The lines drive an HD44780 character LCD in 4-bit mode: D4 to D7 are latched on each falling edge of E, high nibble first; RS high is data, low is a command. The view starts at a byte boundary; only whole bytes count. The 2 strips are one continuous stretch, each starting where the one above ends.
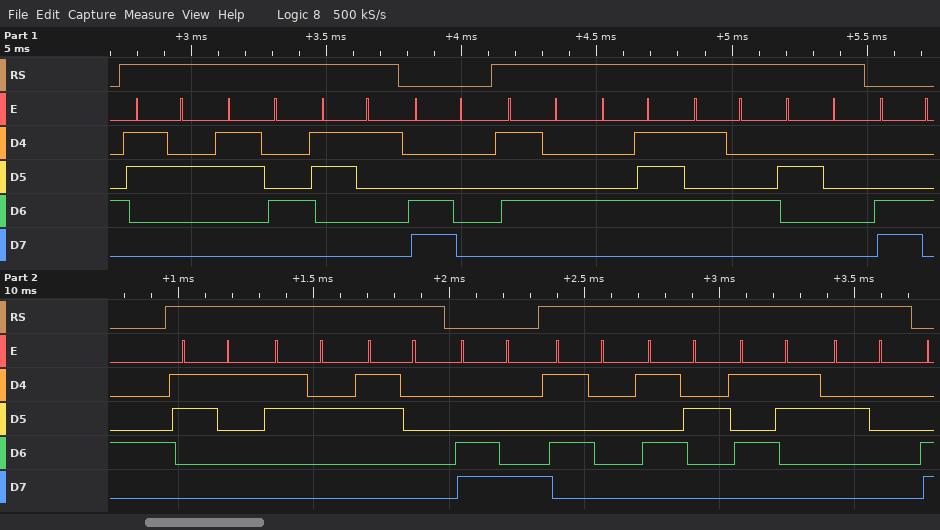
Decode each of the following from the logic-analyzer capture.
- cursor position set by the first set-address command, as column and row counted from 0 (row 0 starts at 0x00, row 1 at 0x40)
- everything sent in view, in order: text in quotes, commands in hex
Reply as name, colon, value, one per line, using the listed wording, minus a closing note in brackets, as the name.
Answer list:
cursor position set by the first set-address command, as column and row counted from 0: column 0, row 1
everything sent in view, in order: text in quotes, commands in hex: "241" 0xC0 "TGT " 0xC4 "120" 0xC8 "PRS "
